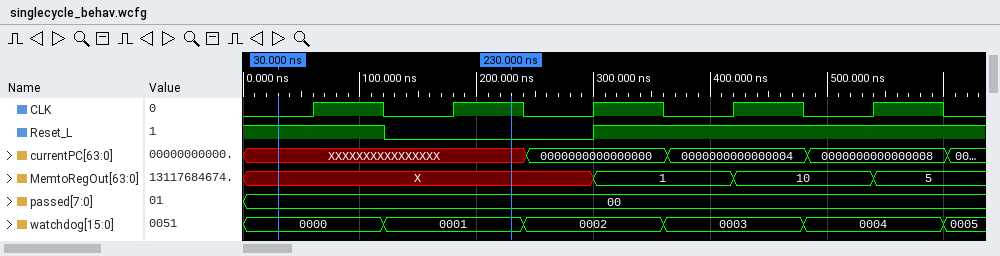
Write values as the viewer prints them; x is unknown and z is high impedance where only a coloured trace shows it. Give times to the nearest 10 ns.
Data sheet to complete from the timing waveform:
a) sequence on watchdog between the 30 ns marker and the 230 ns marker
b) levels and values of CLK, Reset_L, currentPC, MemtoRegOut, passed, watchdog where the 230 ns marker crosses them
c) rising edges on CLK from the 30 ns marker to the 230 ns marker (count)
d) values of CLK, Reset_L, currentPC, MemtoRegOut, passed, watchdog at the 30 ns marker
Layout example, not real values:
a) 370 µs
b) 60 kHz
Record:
a) 0000, 0001
b) CLK=1, Reset_L=0, currentPC=XXXXXXXXXXXXXXXX, MemtoRegOut=X, passed=00, watchdog=0001
c) 2
d) CLK=0, Reset_L=1, currentPC=XXXXXXXXXXXXXXXX, MemtoRegOut=X, passed=00, watchdog=0000
